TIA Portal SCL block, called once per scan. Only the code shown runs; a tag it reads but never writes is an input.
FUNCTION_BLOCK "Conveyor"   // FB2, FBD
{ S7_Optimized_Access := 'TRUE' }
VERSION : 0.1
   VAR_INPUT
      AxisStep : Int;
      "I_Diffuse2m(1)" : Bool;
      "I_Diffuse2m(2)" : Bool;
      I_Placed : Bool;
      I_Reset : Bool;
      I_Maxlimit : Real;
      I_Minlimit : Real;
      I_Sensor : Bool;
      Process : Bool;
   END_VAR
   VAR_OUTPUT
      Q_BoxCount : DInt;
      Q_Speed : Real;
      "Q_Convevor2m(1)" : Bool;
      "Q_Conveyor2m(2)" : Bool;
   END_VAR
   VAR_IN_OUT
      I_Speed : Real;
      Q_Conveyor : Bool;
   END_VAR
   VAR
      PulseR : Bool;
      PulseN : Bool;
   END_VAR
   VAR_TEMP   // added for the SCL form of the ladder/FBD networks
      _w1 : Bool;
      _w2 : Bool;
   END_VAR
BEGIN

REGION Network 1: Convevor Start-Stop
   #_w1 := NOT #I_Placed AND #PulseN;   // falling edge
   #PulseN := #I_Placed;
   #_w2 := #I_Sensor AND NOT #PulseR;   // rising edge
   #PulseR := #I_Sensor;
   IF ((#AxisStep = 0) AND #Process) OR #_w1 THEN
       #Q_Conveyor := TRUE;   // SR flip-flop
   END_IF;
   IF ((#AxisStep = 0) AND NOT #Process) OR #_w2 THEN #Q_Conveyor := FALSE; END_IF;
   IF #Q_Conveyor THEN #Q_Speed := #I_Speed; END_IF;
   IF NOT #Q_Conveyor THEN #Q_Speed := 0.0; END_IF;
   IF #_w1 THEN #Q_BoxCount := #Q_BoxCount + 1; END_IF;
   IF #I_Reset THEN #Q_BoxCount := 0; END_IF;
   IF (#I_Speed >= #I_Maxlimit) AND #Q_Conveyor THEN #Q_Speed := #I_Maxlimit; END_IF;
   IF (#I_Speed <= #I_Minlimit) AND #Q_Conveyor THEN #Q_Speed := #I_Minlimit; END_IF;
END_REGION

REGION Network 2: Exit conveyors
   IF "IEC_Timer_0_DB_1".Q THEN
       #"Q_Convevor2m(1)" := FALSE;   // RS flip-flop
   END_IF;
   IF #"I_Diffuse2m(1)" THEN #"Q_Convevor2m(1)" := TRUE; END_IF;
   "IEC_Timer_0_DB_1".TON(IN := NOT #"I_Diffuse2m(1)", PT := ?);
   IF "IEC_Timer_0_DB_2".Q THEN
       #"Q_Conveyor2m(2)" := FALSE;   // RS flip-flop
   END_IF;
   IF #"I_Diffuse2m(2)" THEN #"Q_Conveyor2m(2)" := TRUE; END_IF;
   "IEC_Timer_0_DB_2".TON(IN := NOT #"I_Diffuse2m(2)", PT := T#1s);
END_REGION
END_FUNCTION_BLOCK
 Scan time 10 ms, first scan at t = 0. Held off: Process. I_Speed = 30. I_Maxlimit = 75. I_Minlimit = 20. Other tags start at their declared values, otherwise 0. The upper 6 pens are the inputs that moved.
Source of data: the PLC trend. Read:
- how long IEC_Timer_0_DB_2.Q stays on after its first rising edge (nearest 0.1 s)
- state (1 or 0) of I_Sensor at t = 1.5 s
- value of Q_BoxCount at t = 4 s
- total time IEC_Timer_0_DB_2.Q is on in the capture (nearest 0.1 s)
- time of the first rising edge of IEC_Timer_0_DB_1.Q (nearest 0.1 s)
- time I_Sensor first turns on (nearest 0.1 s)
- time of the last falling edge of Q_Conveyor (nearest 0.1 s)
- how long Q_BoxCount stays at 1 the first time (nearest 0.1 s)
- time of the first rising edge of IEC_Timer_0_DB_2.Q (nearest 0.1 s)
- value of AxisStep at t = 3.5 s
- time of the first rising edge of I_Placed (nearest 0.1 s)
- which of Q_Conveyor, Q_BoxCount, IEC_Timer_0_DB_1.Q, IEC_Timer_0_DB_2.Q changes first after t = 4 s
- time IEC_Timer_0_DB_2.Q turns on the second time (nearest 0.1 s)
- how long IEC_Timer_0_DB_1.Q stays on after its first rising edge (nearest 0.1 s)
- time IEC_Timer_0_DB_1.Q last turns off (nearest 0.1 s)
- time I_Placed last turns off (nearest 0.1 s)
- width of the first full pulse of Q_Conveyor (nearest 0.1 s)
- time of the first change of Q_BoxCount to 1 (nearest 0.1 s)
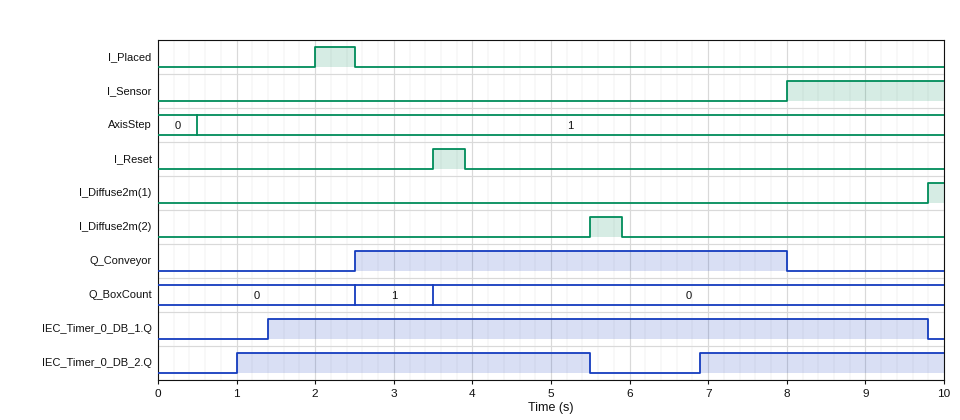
4.5 s
0
0
7.6 s
1.4 s
8.0 s
8.0 s
1.0 s
1.0 s
1
2.0 s
IEC_Timer_0_DB_2.Q
6.9 s
8.4 s
9.8 s
2.5 s
5.5 s
2.5 s
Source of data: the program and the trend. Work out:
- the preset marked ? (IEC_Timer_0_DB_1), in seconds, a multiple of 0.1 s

1.4 s
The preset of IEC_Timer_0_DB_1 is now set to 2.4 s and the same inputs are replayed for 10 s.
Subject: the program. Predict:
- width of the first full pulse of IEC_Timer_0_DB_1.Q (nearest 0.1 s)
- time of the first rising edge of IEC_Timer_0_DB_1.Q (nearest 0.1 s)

7.4 s
2.4 s
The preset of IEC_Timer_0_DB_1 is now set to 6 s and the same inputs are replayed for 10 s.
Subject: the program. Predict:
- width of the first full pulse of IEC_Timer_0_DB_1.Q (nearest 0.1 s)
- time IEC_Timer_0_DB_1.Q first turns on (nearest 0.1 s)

3.8 s
6.0 s
